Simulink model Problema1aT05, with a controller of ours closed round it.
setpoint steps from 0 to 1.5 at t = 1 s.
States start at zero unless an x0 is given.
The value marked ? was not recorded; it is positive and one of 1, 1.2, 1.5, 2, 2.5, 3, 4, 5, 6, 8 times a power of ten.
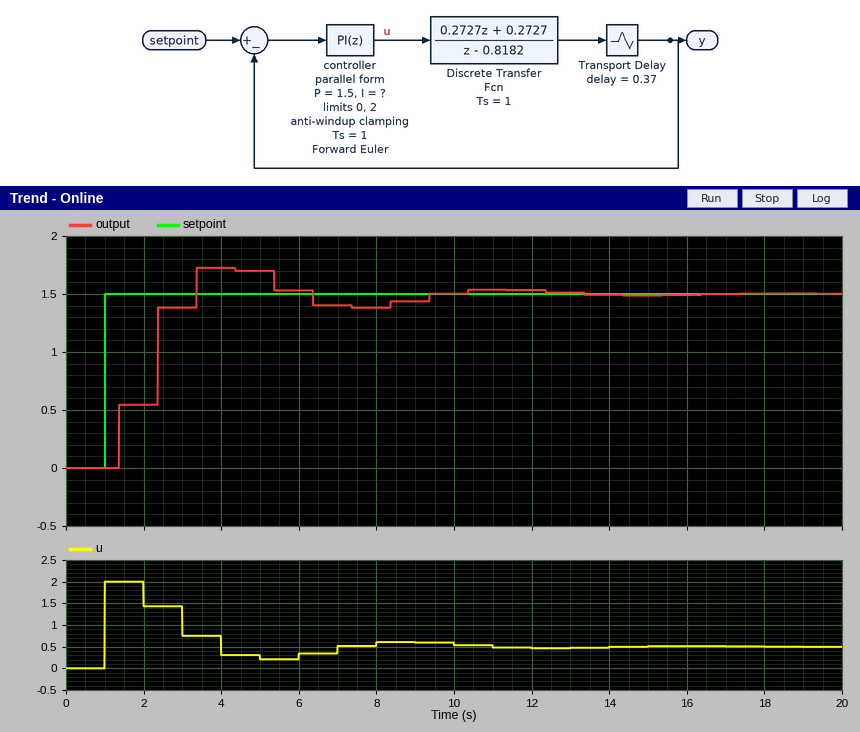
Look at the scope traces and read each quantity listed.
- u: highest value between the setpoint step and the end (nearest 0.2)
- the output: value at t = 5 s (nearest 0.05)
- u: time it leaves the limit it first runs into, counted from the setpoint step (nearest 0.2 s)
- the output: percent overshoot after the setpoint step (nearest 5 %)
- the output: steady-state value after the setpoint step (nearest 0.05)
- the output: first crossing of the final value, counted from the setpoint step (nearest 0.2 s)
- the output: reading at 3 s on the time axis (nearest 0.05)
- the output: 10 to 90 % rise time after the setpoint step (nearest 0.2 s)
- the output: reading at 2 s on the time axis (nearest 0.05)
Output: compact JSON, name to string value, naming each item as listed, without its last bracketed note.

{"u: highest value between the setpoint step and the end": "2.0", "the output: value at t = 5 s": "1.70", "u: time it leaves the limit it first runs into, counted from the setpoint step": "1.0 s", "the output: percent overshoot after the setpoint step": "15 %", "the output: steady-state value after the setpoint step": "1.50", "the output: first crossing of the final value, counted from the setpoint step": "2.4 s", "the output: reading at 3 s on the time axis": "1.40", "the output: 10 to 90 % rise time after the setpoint step": "1.0 s", "the output: reading at 2 s on the time axis": "0.55"}
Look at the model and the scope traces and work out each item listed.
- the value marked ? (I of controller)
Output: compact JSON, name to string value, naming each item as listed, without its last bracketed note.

{"the value marked ?": "0.6"}
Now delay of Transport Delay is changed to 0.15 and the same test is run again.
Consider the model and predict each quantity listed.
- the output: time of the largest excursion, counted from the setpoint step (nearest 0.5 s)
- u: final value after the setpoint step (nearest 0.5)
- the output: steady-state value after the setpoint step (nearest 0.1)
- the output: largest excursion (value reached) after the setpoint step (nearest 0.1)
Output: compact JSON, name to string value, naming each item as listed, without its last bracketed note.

{"the output: time of the largest excursion, counted from the setpoint step": "2.0 s", "u: final value after the setpoint step": "0.5", "the output: steady-state value after the setpoint step": "1.5", "the output: largest excursion (value reached) after the setpoint step": "1.7"}
